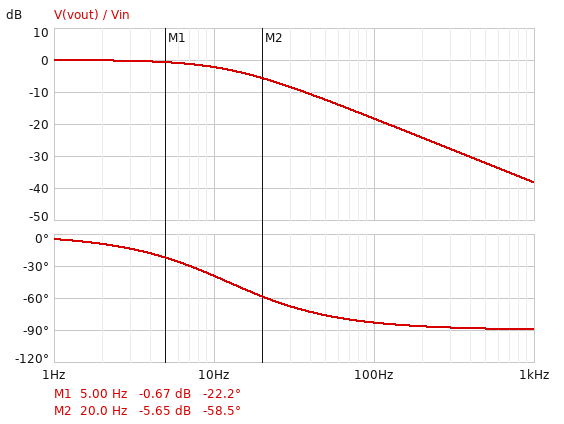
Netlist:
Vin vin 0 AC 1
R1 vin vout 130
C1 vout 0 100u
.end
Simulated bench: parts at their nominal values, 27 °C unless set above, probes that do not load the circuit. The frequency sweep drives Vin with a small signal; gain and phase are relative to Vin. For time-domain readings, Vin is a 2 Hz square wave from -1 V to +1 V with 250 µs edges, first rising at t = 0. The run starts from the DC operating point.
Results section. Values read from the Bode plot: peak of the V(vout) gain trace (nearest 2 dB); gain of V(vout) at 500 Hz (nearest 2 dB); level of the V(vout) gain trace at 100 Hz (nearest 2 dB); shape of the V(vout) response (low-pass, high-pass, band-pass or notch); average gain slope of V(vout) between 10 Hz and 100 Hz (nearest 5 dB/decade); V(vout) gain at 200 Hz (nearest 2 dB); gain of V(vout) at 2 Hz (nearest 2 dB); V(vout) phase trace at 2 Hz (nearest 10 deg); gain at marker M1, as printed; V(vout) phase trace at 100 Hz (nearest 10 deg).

0 dB
-32 dB
-18 dB
low-pass
-15 dB/decade
-24 dB
0 dB
-10 deg
-0.67 dB
-80 deg
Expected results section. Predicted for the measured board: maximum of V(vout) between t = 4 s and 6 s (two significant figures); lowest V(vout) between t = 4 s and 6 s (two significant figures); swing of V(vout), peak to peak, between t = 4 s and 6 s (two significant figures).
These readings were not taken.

1.0 V
-1.0 V
2.0 V
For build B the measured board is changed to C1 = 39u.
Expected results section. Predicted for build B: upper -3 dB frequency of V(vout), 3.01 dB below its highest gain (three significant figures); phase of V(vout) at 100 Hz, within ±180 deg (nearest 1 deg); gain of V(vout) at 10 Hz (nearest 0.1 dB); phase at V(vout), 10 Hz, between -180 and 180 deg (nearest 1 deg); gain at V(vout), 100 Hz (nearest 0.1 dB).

31.4 Hz
-73 deg
-0.4 dB
-18 deg
-10.5 dB
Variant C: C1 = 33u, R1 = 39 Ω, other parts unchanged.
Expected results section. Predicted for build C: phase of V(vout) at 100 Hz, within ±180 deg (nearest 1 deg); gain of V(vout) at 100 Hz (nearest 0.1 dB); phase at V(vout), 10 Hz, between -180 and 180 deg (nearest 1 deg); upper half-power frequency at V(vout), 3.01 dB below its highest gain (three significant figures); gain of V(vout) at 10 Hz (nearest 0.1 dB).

-39 deg
-2.2 dB
-5 deg
124 Hz
0 dB
